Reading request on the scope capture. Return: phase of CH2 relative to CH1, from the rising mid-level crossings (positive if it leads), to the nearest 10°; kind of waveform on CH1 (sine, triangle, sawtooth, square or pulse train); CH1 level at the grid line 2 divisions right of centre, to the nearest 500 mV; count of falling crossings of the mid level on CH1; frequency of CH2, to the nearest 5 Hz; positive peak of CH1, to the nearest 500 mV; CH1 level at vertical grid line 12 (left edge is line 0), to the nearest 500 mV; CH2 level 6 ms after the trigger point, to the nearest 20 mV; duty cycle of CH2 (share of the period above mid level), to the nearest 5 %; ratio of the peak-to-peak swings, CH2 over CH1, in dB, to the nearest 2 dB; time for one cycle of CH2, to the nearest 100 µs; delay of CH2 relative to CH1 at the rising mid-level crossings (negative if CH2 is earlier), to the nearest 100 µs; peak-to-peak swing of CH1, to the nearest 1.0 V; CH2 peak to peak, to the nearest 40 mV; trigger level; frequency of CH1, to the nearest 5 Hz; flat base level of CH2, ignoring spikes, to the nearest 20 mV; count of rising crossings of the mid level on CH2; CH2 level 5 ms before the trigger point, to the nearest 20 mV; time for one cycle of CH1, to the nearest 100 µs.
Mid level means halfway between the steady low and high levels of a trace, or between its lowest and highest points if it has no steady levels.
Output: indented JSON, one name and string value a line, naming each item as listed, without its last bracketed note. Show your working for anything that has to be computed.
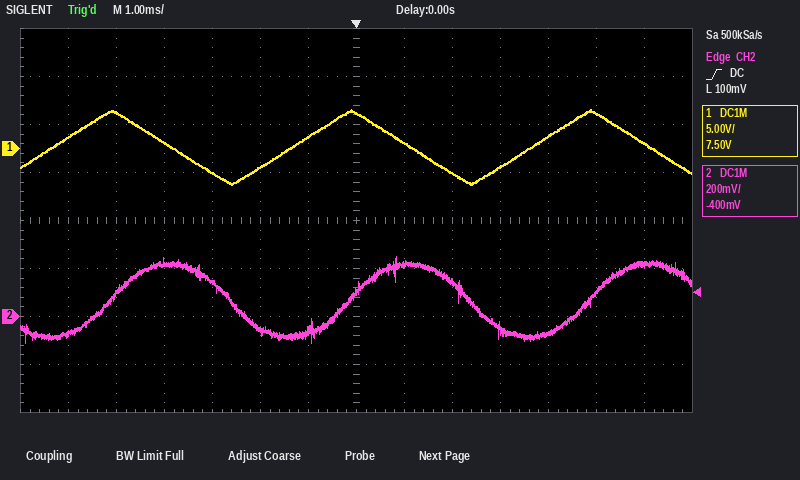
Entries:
{
  "phase of CH2 relative to CH1, from the rising mid-level crossings (positive if it leads), to the nearest 10°": "−360° × (+1.2 ms) / 5.0 ms ≈ -86.4°, so -90° to the nearest 10°",
  "kind of waveform on CH1": "triangle",
  "CH1 level at the grid line 2 divisions right of centre, to the nearest 500 mV": "-2.5 V",
  "count of falling crossings of the mid level on CH1": "3",
  "frequency of CH2, to the nearest 5 Hz": "1 / 5.0 ms ≈ 200 Hz",
  "positive peak of CH1, to the nearest 500 mV": "4.0 V",
  "CH1 level at vertical grid line 12 (left edge is line 0), to the nearest 500 mV": "3.5 V",
  "CH2 level 6 ms after the trigger point, to the nearest 20 mV": "220 mV",
  "duty cycle of CH2 (share of the period above mid level), to the nearest 5 %": "50 %",
  "ratio of the peak-to-peak swings, CH2 over CH1, in dB, to the nearest 2 dB": "20 log10(360 mV / 8.0 V) ≈ -26.9 dB, so -26 dB to the nearest 2 dB",
  "time for one cycle of CH2, to the nearest 100 µs": "5.0 ms",
  "delay of CH2 relative to CH1 at the rising mid-level crossings (negative if CH2 is earlier), to the nearest 100 µs": "+1.2 ms",
  "peak-to-peak swing of CH1, to the nearest 1.0 V": "8.0 V",
  "CH2 peak to peak, to the nearest 40 mV": "360 mV",
  "trigger level": "100 mV",
  "frequency of CH1, to the nearest 5 Hz": "1 / 5.0 ms ≈ 200 Hz",
  "flat base level of CH2, ignoring spikes, to the nearest 20 mV": "-80 mV",
  "count of rising crossings of the mid level on CH2": "3",
  "CH2 level 5 ms before the trigger point, to the nearest 20 mV": "100 mV",
  "time for one cycle of CH1, to the nearest 100 µs": "5.0 ms"
}
